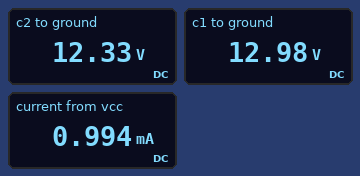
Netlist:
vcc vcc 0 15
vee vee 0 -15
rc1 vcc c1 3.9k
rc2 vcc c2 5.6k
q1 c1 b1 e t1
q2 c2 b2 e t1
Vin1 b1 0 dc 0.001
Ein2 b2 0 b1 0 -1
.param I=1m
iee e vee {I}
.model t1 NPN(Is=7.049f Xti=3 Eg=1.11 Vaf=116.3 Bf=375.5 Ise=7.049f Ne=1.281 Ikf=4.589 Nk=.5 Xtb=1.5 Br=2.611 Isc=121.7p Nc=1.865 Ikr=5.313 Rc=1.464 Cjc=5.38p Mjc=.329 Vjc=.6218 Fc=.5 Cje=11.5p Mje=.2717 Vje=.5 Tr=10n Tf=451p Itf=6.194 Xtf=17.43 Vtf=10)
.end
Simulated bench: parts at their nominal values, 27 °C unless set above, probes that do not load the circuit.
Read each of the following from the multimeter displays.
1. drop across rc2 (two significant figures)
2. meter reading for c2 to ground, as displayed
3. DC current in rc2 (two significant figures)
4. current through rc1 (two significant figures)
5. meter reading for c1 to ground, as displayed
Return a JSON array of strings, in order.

["2.7 V", "12.33 V", "480 µA", "520 µA", "12.98 V"]
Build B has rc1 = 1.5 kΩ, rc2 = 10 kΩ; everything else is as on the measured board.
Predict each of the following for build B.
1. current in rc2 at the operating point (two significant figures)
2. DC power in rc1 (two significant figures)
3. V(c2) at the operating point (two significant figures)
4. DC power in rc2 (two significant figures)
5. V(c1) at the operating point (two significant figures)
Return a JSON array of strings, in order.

["470 µA", "410 µW", "10 V", "2.2 mW", "14 V"]
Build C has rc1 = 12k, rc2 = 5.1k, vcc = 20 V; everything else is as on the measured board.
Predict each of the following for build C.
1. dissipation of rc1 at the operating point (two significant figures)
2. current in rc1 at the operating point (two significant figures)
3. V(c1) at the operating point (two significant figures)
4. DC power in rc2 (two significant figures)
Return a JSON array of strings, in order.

["3.1 mW", "510 µA", "14 V", "1.2 mW"]
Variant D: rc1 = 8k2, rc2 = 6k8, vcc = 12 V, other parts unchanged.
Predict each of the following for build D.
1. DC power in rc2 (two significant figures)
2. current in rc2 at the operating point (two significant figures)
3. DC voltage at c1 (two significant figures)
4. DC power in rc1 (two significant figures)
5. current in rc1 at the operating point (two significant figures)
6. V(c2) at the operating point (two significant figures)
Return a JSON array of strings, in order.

["1.6 mW", "480 µA", "7.8 V", "2.2 mW", "510 µA", "8.7 V"]
